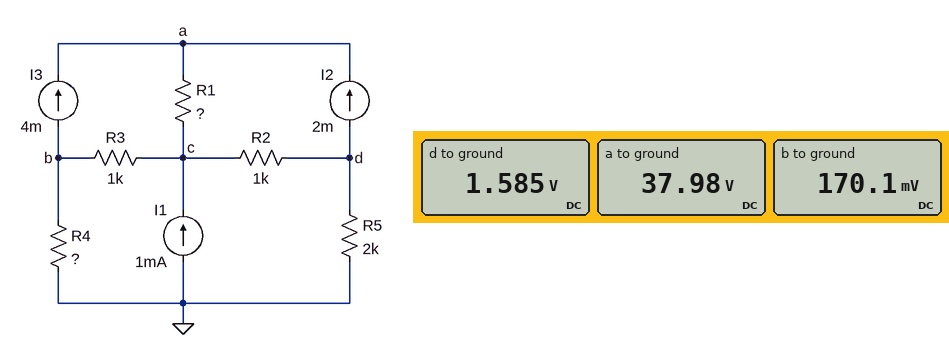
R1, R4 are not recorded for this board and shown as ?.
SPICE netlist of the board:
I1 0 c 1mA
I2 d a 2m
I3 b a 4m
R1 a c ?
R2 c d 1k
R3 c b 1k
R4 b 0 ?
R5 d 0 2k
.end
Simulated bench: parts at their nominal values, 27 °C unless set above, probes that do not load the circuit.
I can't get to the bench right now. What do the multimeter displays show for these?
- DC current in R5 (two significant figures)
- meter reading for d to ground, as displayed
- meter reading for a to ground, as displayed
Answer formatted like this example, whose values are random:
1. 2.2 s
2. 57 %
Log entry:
1. 790 µA
2. 1.585 V
3. 37.98 V
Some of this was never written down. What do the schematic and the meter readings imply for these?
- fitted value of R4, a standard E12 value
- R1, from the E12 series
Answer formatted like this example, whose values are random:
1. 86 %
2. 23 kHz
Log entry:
1. 820 Ω
2. 5.6 kΩ
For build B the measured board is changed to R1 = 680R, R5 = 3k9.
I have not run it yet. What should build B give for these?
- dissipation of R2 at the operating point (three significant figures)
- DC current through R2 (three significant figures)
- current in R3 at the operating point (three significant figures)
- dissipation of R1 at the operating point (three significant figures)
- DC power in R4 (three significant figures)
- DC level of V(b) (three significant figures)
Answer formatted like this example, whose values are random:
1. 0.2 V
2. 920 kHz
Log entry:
1. 6.60 mW
2. 2.57 mA
3. 4.43 mA
4. 24.5 mW
5. 153 µW
6. 354 mV
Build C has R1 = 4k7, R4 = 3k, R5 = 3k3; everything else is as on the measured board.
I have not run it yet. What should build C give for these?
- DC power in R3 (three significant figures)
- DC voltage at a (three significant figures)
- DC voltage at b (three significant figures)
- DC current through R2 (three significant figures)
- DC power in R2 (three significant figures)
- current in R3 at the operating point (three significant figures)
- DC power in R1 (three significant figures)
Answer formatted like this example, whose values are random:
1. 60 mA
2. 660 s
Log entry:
1. 18.3 mW
2. 33.3 V
3. 831 mV
4. 2.72 mA
5. 7.41 mW
6. 4.28 mA
7. 169 mW
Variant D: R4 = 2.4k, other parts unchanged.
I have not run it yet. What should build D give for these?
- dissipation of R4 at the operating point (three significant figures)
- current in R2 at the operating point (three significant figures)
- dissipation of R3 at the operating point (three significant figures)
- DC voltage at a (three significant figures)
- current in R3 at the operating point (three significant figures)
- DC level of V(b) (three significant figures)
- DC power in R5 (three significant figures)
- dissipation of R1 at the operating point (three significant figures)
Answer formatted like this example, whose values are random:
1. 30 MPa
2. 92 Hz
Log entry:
1. 58.6 µW
2. 2.84 mA
3. 17.3 mW
4. 38.1 V
5. 4.16 mA
6. 375 mV
7. 1.42 mW
8. 202 mW
